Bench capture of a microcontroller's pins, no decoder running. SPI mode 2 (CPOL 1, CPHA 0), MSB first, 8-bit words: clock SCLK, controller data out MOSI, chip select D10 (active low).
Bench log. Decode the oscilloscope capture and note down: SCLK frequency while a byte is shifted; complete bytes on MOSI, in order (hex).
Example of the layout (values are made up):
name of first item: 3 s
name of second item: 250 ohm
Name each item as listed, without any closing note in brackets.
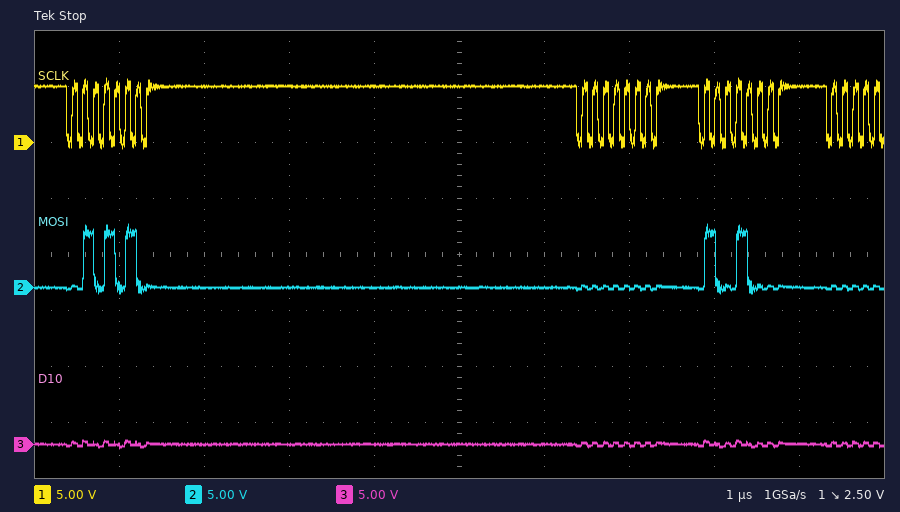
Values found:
SCLK frequency while a byte is shifted: 8 MHz
complete bytes on MOSI, in order: 2A 00 48
